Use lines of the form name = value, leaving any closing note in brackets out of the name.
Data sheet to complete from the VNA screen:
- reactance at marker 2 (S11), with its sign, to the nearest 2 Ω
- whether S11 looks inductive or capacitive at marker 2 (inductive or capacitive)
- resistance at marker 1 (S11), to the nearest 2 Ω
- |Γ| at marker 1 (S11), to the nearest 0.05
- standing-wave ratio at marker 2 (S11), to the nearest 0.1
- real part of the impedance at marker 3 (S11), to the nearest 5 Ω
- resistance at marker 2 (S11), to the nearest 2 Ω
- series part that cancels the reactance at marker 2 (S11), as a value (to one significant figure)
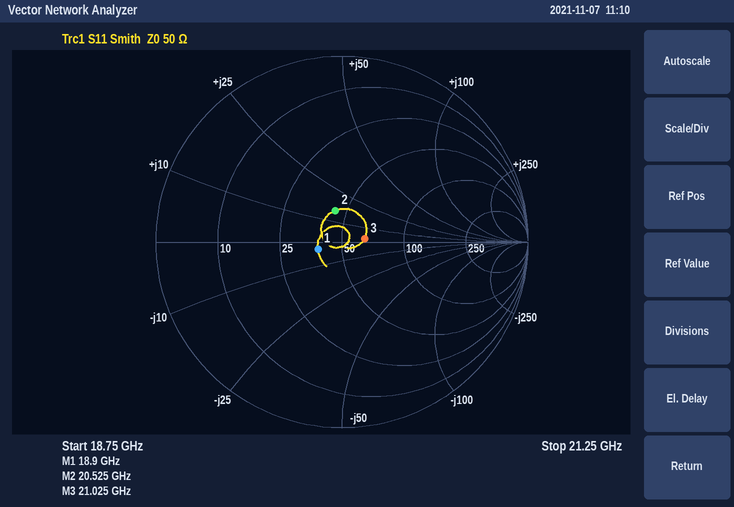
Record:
reactance at marker 2 (S11), with its sign, to the nearest 2 Ω = +16 Ω
whether S11 looks inductive or capacitive at marker 2 = inductive
resistance at marker 1 (S11), to the nearest 2 Ω = 38 Ω
|Γ| at marker 1 (S11), to the nearest 0.05 = 0.15
standing-wave ratio at marker 2 (S11), to the nearest 0.1 = 1.4
real part of the impedance at marker 3 (S11), to the nearest 5 Ω = 65 Ω
resistance at marker 2 (S11), to the nearest 2 Ω = 44 Ω
series part that cancels the reactance at marker 2 (S11), as a value = 500 fF
